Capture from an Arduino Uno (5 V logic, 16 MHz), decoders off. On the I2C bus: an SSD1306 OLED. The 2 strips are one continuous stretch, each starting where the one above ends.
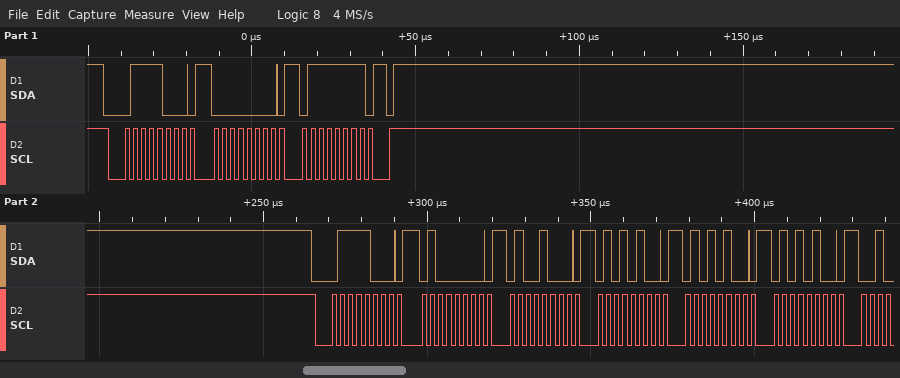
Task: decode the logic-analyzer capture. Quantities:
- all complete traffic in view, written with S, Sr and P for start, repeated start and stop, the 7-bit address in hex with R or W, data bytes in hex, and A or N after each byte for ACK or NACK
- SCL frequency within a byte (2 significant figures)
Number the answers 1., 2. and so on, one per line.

1. S 3CW A 00 A 7F A P S 3CW A 40 A 48 A 54 A 54 A 54 A
2. 400 kHz
